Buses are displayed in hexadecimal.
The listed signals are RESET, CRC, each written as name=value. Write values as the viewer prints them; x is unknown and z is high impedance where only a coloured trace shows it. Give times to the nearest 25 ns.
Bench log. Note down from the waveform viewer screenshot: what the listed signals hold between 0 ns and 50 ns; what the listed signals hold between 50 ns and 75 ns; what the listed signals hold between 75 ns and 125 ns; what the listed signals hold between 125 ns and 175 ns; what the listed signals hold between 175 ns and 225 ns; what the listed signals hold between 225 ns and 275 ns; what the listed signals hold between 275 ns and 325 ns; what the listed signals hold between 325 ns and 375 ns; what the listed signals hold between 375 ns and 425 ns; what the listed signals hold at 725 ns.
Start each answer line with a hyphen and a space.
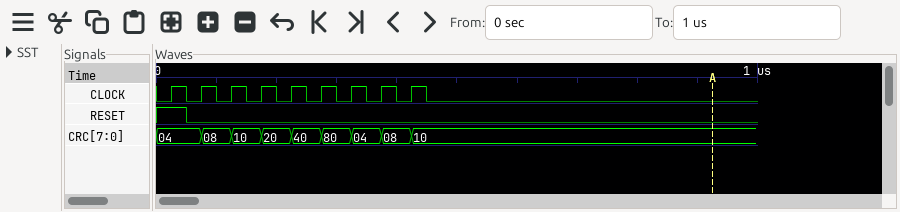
- RESET=1, CRC=04
- RESET=0, CRC=04
- RESET=0, CRC=08
- RESET=0, CRC=10
- RESET=0, CRC=20
- RESET=0, CRC=40
- RESET=0, CRC=80
- RESET=0, CRC=04
- RESET=0, CRC=08
- RESET=0, CRC=10
